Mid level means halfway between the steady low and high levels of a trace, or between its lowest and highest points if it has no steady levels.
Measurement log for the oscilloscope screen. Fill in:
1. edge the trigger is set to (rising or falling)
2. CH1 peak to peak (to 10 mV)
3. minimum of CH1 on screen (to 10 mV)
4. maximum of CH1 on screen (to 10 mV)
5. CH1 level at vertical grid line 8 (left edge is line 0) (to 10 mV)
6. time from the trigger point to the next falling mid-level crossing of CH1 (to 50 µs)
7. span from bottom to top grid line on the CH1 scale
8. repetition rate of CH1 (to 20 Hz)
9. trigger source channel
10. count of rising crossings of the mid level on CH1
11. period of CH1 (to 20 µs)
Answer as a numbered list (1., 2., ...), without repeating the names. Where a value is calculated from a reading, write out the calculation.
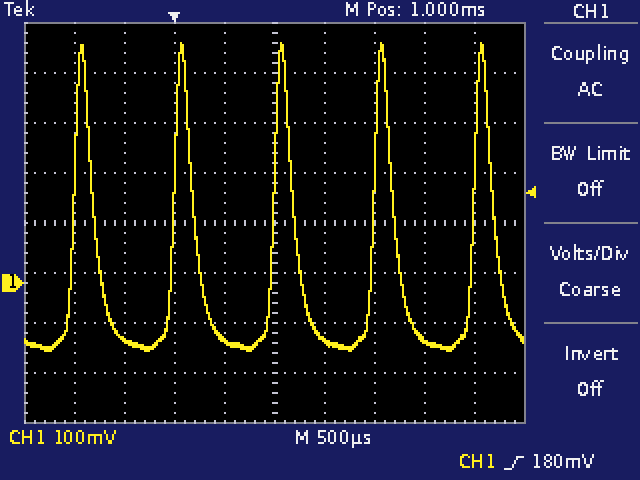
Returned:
1. rising
2. 480 mV − (-140 mV) = 620 mV
3. -140 mV
4. 480 mV
5. -110 mV
6. 200 µs
7. 800 mV
8. 1 / 1.00 ms ≈ 1.00 kHz
9. CH1
10. 5
11. 1.00 ms
